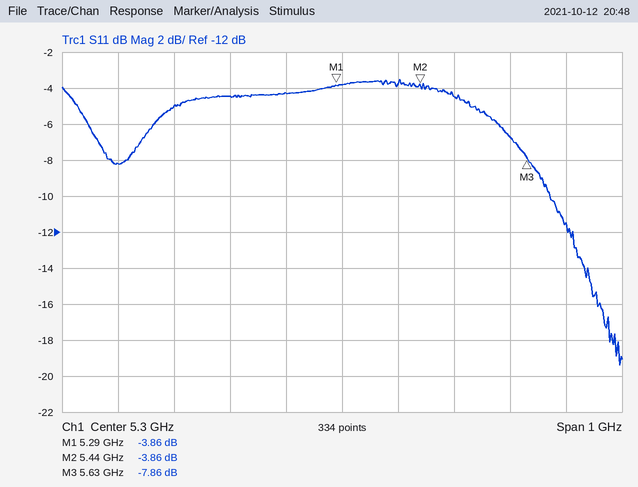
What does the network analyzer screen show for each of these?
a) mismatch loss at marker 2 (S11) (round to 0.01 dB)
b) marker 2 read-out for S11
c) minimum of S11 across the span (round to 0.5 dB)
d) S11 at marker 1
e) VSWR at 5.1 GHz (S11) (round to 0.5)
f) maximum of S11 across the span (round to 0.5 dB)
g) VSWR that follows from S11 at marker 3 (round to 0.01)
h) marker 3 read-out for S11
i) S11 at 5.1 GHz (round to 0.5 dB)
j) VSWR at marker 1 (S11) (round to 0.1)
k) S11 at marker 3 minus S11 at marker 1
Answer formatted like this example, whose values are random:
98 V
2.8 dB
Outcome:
2.30 dB
-3.86 dB
-19.5 dB
-3.86 dB
4.0
-3.5 dB
2.36
-7.86 dB
-4.5 dB
4.6
-4.00 dB
